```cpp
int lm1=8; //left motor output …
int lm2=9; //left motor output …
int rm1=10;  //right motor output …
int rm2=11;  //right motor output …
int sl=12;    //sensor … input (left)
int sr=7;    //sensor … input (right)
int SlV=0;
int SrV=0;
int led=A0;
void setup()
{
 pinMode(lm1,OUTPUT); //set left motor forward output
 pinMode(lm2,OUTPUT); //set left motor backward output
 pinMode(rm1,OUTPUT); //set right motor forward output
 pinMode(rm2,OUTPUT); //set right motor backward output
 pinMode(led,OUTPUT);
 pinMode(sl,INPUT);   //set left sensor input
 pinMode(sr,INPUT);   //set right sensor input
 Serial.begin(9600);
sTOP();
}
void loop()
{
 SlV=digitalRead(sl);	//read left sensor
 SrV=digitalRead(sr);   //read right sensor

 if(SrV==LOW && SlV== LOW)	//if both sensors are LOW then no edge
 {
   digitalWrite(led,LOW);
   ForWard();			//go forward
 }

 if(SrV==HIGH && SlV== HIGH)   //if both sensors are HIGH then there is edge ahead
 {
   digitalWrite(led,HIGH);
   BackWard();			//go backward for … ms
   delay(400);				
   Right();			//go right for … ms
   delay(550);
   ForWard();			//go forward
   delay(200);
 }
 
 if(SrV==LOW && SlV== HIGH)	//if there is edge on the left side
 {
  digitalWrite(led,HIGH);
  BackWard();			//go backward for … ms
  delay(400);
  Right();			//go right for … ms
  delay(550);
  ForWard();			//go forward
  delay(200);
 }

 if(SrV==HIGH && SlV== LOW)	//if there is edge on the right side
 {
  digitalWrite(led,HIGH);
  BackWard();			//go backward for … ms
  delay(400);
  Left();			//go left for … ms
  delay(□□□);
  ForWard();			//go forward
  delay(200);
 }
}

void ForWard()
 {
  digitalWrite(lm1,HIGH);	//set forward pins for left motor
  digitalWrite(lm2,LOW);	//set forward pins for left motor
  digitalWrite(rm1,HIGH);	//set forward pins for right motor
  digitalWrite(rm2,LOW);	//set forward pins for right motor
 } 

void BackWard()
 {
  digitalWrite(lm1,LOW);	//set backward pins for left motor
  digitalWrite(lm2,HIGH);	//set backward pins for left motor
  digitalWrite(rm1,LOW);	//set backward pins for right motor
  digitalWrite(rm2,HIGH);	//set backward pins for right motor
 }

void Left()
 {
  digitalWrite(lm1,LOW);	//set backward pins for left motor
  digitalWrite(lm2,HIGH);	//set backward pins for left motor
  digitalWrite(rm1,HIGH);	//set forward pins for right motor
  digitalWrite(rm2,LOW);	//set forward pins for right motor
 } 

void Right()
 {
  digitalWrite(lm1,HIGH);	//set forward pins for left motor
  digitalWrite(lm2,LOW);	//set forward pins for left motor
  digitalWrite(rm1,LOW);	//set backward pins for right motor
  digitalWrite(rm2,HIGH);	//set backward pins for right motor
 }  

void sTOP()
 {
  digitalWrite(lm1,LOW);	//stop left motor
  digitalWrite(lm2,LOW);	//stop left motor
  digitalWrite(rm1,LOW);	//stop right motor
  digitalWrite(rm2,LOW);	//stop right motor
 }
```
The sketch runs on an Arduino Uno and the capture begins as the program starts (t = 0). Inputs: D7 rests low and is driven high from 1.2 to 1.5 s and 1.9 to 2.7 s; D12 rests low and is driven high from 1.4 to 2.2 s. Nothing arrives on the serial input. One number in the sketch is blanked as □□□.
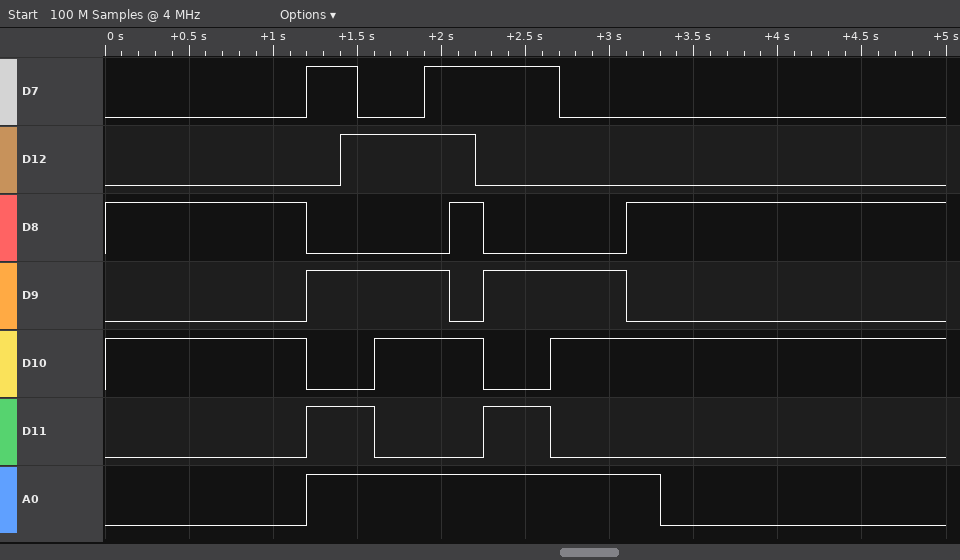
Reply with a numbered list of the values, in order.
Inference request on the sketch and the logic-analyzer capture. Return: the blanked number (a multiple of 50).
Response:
1. 450
